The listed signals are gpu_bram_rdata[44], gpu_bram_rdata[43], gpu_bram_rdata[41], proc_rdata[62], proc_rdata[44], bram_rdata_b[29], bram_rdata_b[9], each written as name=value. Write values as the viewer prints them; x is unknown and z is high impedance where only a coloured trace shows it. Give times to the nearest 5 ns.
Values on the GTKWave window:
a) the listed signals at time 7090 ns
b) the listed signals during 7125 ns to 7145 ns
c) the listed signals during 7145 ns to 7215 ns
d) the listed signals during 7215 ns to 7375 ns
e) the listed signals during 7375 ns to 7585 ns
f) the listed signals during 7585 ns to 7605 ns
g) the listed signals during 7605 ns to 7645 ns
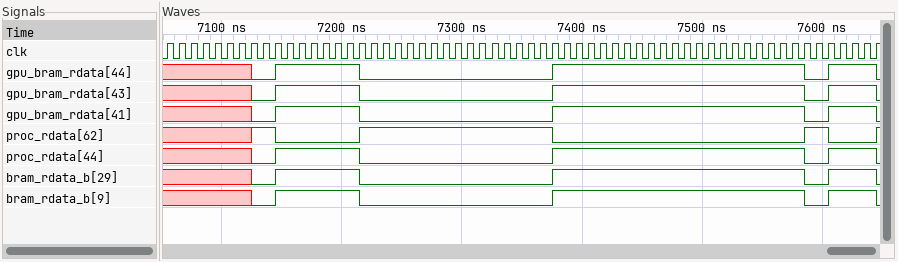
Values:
gpu_bram_rdata[44]=x, gpu_bram_rdata[43]=x, gpu_bram_rdata[41]=x, proc_rdata[62]=x, proc_rdata[44]=x, bram_rdata_b[29]=x, bram_rdata_b[9]=x
gpu_bram_rdata[44]=0, gpu_bram_rdata[43]=0, gpu_bram_rdata[41]=0, proc_rdata[62]=1, proc_rdata[44]=0, bram_rdata_b[29]=0, bram_rdata_b[9]=0
gpu_bram_rdata[44]=1, gpu_bram_rdata[43]=1, gpu_bram_rdata[41]=1, proc_rdata[62]=0, proc_rdata[44]=1, bram_rdata_b[29]=1, bram_rdata_b[9]=1
gpu_bram_rdata[44]=0, gpu_bram_rdata[43]=0, gpu_bram_rdata[41]=0, proc_rdata[62]=1, proc_rdata[44]=0, bram_rdata_b[29]=0, bram_rdata_b[9]=0
gpu_bram_rdata[44]=1, gpu_bram_rdata[43]=1, gpu_bram_rdata[41]=1, proc_rdata[62]=0, proc_rdata[44]=1, bram_rdata_b[29]=1, bram_rdata_b[9]=1
gpu_bram_rdata[44]=0, gpu_bram_rdata[43]=0, gpu_bram_rdata[41]=0, proc_rdata[62]=1, proc_rdata[44]=0, bram_rdata_b[29]=0, bram_rdata_b[9]=0
gpu_bram_rdata[44]=1, gpu_bram_rdata[43]=1, gpu_bram_rdata[41]=1, proc_rdata[62]=0, proc_rdata[44]=1, bram_rdata_b[29]=1, bram_rdata_b[9]=1
